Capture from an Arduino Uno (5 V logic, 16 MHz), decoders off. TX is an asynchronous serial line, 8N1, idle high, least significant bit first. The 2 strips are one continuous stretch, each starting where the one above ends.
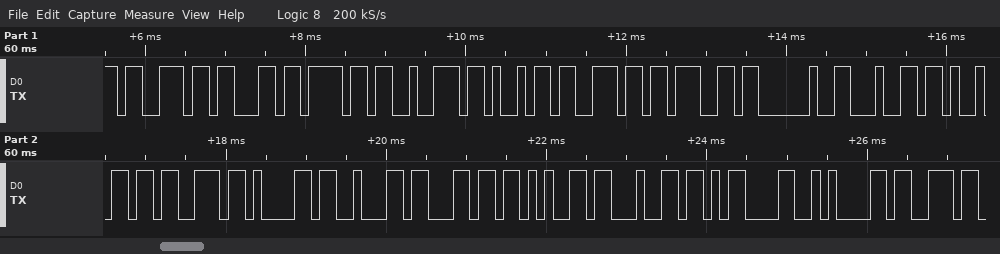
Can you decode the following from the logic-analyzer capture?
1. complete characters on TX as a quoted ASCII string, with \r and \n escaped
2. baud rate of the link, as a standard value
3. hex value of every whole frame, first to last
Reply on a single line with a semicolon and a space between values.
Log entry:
"scoring disabled\r\ns"; 9600 baud; 73 63 6F 72 69 6E 67 20 64 69 73 61 62 6C 65 64 0D 0A 73
